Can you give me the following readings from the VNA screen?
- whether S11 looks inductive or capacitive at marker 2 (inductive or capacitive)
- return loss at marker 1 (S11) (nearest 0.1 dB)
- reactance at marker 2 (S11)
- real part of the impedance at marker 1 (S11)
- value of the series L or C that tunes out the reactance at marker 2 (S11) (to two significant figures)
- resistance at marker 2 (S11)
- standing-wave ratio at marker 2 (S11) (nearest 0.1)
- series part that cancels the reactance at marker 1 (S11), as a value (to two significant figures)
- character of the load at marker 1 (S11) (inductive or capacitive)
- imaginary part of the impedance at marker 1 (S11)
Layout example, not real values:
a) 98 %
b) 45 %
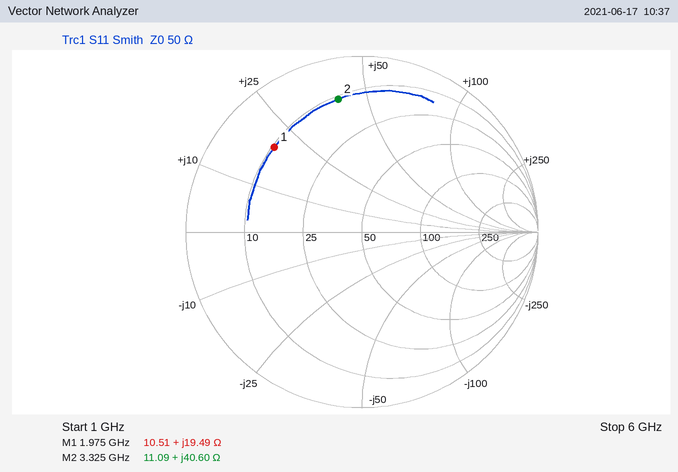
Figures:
a) inductive
b) 3.2 dB
c) +40.60 Ω
d) 10.51 Ω
e) 1.2 pF
f) 11.09 Ω
g) 7.6
h) 4.1 pF
i) inductive
j) +19.49 Ω
